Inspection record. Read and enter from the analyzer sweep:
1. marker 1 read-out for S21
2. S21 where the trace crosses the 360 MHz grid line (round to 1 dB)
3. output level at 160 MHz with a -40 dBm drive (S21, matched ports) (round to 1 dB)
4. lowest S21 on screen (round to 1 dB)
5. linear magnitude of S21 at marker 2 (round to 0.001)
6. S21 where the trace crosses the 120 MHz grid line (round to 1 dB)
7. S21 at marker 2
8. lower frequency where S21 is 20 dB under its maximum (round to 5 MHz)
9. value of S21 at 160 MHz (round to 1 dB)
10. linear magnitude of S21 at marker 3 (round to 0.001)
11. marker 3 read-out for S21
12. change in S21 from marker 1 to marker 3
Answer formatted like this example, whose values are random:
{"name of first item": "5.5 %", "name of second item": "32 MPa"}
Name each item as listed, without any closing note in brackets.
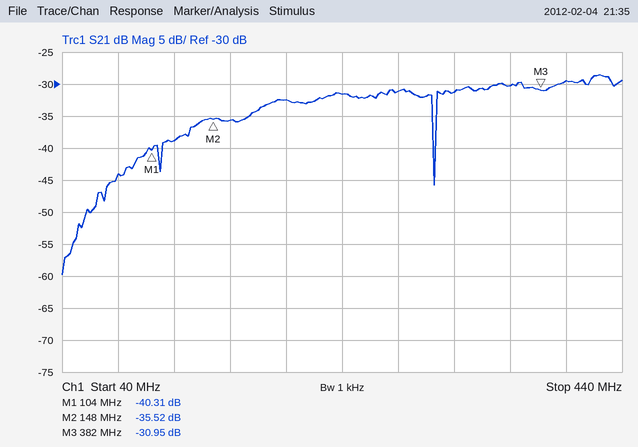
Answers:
{"marker 1 read-out for S21": "-40.31 dB", "S21 where the trace crosses the 360 MHz grid line": "-30 dB", "output level at 160 MHz with a -40 dBm drive (S21, matched ports)": "-76 dBm", "lowest S21 on screen": "-60 dB", "linear magnitude of S21 at marker 2": "0.017", "S21 where the trace crosses the 120 MHz grid line": "-39 dB", "S21 at marker 2": "-35.52 dB", "lower frequency where S21 is 20 dB under its maximum": "65 MHz", "value of S21 at 160 MHz": "-36 dB", "linear magnitude of S21 at marker 3": "0.028", "marker 3 read-out for S21": "-30.95 dB", "change in S21 from marker 1 to marker 3": "9.36 dB"}
